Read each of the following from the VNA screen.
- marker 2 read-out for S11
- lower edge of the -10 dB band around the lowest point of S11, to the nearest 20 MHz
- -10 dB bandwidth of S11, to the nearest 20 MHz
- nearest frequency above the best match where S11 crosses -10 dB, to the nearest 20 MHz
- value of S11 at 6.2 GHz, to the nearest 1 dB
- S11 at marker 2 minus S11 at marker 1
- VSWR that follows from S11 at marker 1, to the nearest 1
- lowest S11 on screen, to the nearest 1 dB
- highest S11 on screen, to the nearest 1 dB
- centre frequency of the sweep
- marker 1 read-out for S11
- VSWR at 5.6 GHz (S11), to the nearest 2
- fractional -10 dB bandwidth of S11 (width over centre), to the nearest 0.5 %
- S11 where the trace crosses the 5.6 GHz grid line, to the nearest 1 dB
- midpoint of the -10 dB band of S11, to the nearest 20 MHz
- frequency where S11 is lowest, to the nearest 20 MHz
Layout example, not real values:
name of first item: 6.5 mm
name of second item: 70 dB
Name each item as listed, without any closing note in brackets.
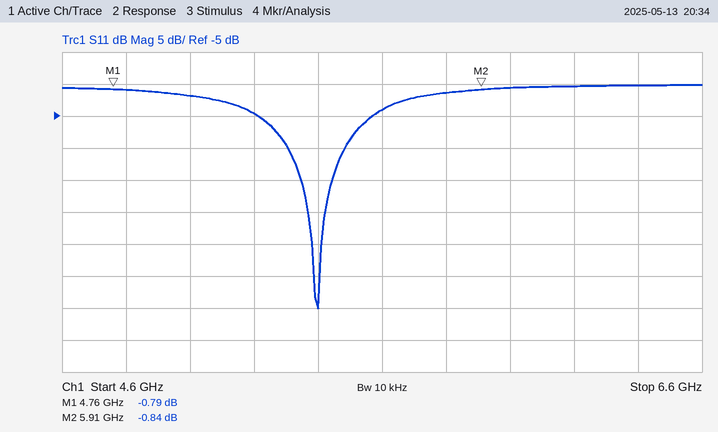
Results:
marker 2 read-out for S11: -0.84 dB
lower edge of the -10 dB band around the lowest point of S11, to the nearest 20 MHz: 5.30 GHz
-10 dB bandwidth of S11, to the nearest 20 MHz: 180 MHz
nearest frequency above the best match where S11 crosses -10 dB, to the nearest 20 MHz: 5.48 GHz
value of S11 at 6.2 GHz, to the nearest 1 dB: 0 dB
S11 at marker 2 minus S11 at marker 1: -0.05 dB
VSWR that follows from S11 at marker 1, to the nearest 1: 22
lowest S11 on screen, to the nearest 1 dB: -35 dB
highest S11 on screen, to the nearest 1 dB: 0 dB
centre frequency of the sweep: 5.6 GHz
marker 1 read-out for S11: -0.79 dB
VSWR at 5.6 GHz (S11), to the nearest 2: 4
fractional -10 dB bandwidth of S11 (width over centre), to the nearest 0.5 %: 3.5 %
S11 where the trace crosses the 5.6 GHz grid line, to the nearest 1 dB: -4 dB
midpoint of the -10 dB band of S11, to the nearest 20 MHz: 5.40 GHz
frequency where S11 is lowest, to the nearest 20 MHz: 5.40 GHz
